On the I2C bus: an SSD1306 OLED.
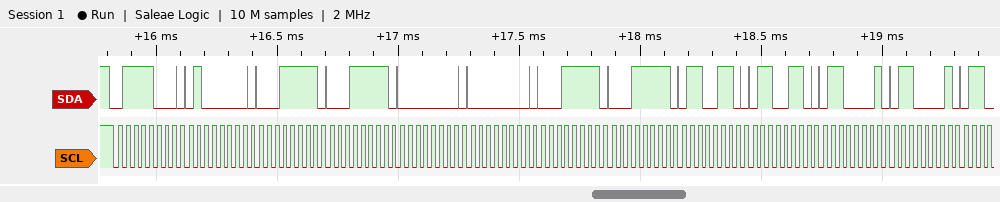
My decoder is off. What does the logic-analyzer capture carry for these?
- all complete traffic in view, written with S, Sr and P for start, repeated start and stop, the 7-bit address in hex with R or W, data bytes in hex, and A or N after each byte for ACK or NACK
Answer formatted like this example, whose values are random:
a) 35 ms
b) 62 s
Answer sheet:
a) S 3CW A 40 A 1F A 1F A 00 A 00 A 1F A 1F A 66 A 66 A 61 A 61 A
